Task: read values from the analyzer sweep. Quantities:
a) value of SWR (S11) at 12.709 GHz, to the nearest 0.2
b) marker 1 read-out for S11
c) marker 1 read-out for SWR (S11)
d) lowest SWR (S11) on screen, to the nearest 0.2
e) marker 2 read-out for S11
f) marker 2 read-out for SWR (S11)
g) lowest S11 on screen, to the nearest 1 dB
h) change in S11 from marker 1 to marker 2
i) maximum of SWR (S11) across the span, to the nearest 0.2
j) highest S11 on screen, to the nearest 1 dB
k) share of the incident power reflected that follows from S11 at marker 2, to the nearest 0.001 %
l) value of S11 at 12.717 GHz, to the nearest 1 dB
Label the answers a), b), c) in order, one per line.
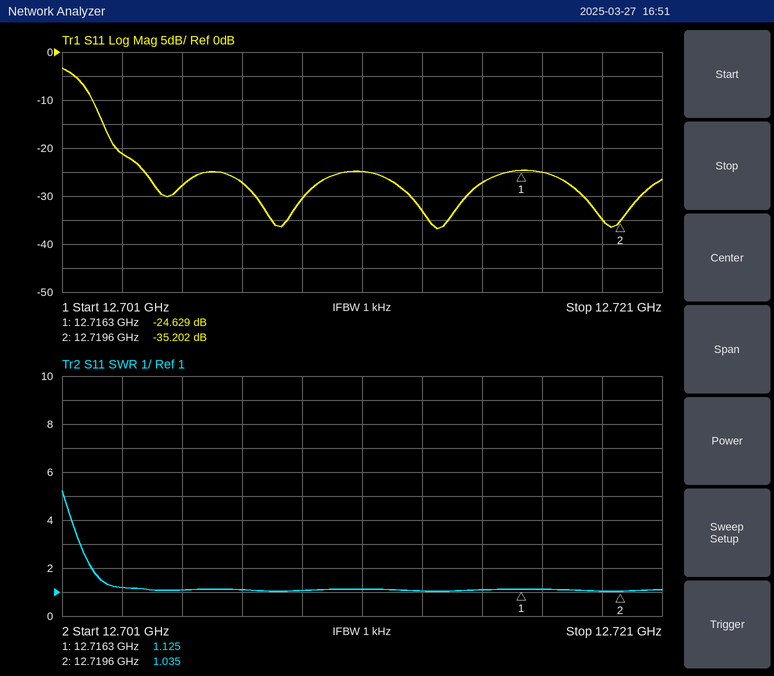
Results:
a) 1.0
b) -24.629 dB
c) 1.125
d) 1.0
e) -35.202 dB
f) 1.035
g) -37 dB
h) -10.573 dB
i) 5.2
j) -3 dB
k) 0.030 %
l) -25 dB
